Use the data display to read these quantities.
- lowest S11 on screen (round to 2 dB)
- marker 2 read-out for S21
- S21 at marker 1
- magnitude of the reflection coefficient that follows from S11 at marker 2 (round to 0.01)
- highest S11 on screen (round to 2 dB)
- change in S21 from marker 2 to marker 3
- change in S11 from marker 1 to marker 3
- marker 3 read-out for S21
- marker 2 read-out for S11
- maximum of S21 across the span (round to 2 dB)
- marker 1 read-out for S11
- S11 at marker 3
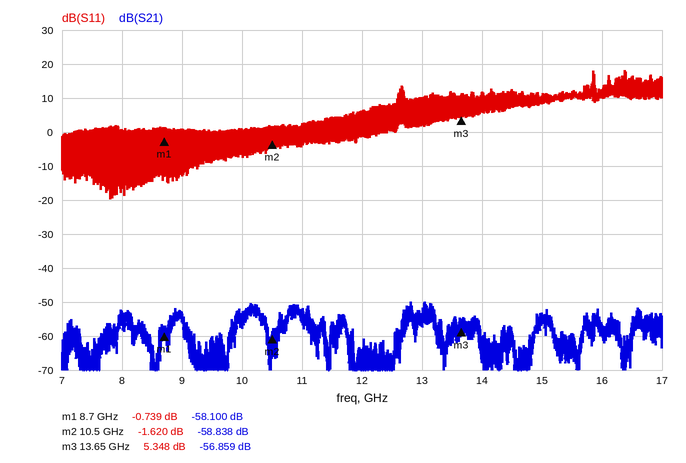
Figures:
-20 dB
-58.838 dB
-58.100 dB
0.83
18 dB
1.979 dB
6.087 dB
-56.859 dB
-1.620 dB
-50 dB
-0.739 dB
5.348 dB
